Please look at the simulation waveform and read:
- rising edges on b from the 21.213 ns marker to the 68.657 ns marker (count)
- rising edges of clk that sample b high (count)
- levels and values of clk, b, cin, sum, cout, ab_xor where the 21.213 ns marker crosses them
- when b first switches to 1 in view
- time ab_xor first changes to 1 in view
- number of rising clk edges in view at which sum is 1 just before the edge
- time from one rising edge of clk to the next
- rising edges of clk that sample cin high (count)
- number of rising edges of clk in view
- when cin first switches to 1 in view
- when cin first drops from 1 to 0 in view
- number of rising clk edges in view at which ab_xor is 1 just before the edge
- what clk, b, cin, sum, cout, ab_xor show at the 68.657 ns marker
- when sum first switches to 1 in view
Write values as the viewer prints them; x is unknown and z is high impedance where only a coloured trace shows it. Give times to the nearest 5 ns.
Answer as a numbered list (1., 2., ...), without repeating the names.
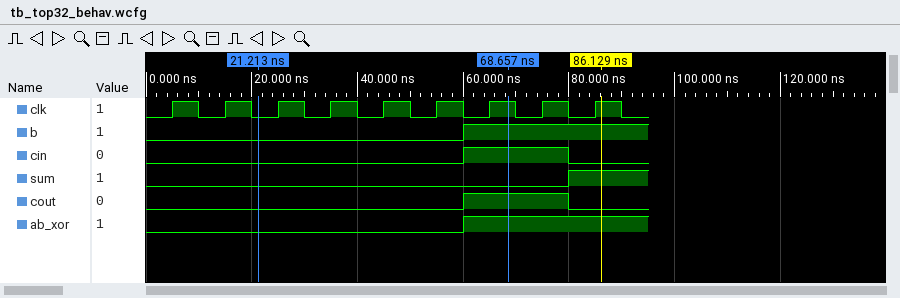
1. 1
2. 3
3. clk=0, b=0, cin=0, sum=0, cout=0, ab_xor=0
4. 60 ns
5. 60 ns
6. 1
7. 10 ns
8. 2
9. 9
10. 60 ns
11. 80 ns
12. 3
13. clk=1, b=1, cin=1, sum=0, cout=1, ab_xor=1
14. 80 ns
